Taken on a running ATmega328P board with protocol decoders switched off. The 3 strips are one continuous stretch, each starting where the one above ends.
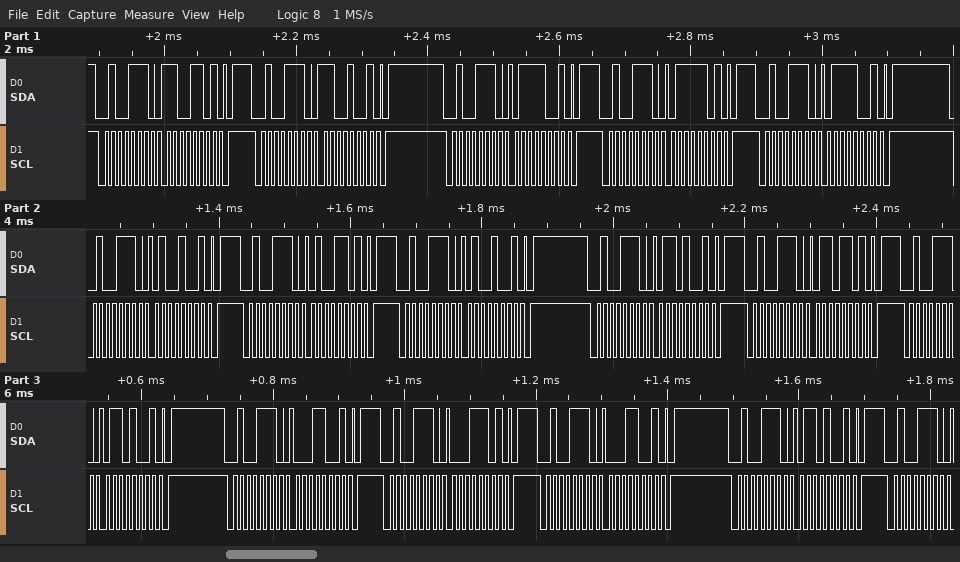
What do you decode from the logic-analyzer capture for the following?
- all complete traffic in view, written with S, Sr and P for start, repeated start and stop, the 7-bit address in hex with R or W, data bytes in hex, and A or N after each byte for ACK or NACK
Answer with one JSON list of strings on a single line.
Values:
["S 27W A CD A P S 27W A C9 A P S 27W A 79 A P S 27W A 7D A P S 27W A 79 A P S 27W A 49 A P S 27W A 4D A P S 27W A 49 A P S 27W A 69 A P S 27W A 6D A P S 27W A 69 A P S 27W A 19 A P S 27W A 1D A P S 27W A 19 A P S 27W A 69 A P S 27W A"]
